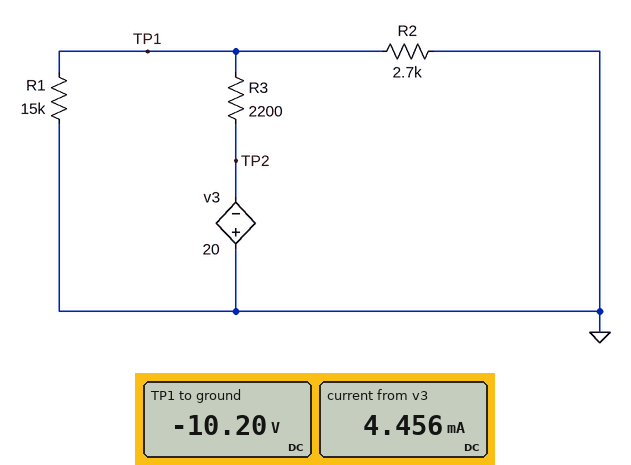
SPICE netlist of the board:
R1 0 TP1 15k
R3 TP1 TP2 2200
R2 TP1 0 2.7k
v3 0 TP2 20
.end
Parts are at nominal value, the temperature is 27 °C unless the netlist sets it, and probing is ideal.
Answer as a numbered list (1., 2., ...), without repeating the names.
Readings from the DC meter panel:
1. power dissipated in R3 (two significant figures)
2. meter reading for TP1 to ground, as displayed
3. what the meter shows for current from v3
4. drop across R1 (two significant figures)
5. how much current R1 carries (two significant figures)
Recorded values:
1. 44 mW
2. -10.20 V
3. 4.456 mA
4. 10 V
5. 680 µA
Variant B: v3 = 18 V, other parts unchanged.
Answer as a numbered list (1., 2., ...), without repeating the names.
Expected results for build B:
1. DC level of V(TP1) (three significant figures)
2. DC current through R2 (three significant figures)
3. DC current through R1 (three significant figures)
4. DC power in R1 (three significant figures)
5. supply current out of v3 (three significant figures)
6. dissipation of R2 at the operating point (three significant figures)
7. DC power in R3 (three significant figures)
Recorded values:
1. -9.18 V
2. 3.40 mA
3. 612 µA
4. 5.61 mW
5. 4.01 mA
6. 31.2 mW
7. 35.4 mW
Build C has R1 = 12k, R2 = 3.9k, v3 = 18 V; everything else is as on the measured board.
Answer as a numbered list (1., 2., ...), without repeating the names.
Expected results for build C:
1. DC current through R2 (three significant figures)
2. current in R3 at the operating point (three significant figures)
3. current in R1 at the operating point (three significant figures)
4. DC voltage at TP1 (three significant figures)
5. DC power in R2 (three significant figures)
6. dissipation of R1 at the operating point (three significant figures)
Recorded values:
1. 2.64 mA
2. 3.50 mA
3. 858 µA
4. -10.3 V
5. 27.2 mW
6. 8.84 mW
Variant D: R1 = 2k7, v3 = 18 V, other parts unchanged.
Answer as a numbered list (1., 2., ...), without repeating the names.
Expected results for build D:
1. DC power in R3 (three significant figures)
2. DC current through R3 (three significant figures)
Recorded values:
1. 56.6 mW
2. 5.07 mA
